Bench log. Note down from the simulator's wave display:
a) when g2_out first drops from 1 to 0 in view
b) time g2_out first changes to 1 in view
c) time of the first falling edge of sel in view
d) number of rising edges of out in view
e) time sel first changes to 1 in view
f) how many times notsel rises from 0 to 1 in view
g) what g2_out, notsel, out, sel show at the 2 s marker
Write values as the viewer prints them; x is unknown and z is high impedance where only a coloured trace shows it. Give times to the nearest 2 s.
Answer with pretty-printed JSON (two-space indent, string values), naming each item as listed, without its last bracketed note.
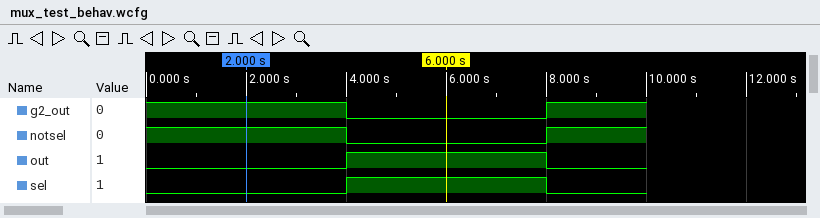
{
  "when g2_out first drops from 1 to 0 in view": "4 s",
  "time g2_out first changes to 1 in view": "8 s",
  "time of the first falling edge of sel in view": "8 s",
  "number of rising edges of out in view": "1",
  "time sel first changes to 1 in view": "4 s",
  "how many times notsel rises from 0 to 1 in view": "1",
  "what g2_out, notsel, out, sel show at the 2 s marker": "g2_out=1, notsel=1, out=0, sel=0"
}
